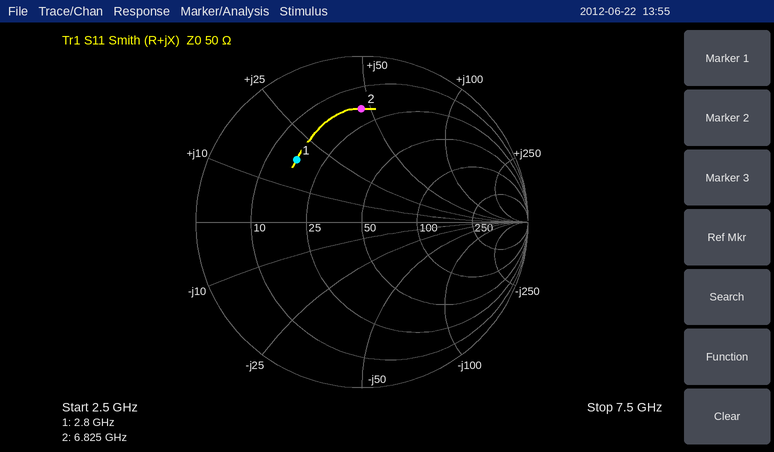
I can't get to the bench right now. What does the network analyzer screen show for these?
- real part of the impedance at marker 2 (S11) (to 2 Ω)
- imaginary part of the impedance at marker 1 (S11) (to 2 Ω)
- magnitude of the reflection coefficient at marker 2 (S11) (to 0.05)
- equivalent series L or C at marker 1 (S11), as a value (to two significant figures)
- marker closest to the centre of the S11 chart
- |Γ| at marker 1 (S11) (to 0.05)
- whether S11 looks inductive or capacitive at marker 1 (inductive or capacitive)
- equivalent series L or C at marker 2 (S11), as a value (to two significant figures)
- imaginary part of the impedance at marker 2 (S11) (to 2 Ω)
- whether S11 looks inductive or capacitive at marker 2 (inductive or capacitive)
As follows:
18 Ω
+18 Ω
0.70
1.0 nH
marker 1
0.55
inductive
1.1 nH
+46 Ω
inductive
